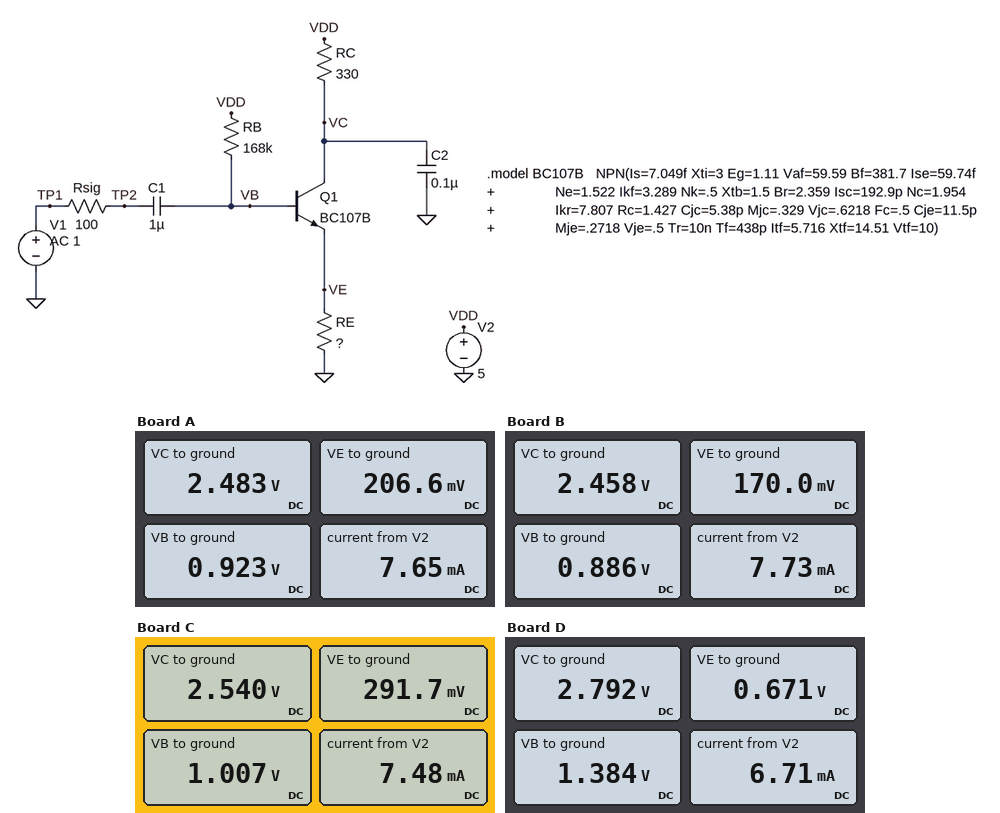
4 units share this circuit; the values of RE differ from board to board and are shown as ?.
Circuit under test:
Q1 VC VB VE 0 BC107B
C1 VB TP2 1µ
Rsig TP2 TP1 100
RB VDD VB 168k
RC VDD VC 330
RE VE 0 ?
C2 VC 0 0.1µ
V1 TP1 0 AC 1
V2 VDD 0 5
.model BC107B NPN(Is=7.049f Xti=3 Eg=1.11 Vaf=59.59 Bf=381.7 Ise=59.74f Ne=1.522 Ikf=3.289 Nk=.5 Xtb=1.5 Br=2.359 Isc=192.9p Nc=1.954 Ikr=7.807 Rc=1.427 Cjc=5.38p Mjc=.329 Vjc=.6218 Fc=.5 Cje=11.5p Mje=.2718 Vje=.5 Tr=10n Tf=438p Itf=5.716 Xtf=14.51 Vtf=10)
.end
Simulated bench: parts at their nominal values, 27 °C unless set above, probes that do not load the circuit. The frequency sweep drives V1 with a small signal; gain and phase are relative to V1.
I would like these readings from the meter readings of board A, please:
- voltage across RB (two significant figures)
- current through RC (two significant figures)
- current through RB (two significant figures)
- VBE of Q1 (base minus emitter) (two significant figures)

4.1 V
7.6 mA
24 µA
720 mV
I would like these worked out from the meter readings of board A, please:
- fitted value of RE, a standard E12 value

27 Ω
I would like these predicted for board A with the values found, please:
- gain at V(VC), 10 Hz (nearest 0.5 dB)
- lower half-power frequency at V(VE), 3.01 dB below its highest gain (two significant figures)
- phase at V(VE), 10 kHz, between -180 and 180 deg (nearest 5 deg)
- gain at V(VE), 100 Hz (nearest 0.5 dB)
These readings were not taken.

14.5 dB
17 Hz
0 deg
-1.5 dB
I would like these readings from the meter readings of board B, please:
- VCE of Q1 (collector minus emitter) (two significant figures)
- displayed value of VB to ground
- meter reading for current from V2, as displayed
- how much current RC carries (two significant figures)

2.3 V
0.886 V
7.73 mA
7.7 mA
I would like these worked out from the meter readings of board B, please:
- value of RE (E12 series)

22 Ω
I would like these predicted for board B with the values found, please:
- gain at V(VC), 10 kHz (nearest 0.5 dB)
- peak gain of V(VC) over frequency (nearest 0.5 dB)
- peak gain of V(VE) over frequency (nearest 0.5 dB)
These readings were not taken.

15.0 dB
22.0 dB
-1.5 dB
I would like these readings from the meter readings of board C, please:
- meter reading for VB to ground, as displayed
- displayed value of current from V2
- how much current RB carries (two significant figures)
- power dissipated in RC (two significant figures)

1.007 V
7.48 mA
24 µA
18 mW
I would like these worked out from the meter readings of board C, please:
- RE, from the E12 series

39 Ω
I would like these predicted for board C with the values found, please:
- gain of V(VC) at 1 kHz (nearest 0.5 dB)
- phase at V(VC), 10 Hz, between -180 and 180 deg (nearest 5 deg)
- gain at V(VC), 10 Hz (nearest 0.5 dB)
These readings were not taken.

17.5 dB
-130 deg
13.5 dB
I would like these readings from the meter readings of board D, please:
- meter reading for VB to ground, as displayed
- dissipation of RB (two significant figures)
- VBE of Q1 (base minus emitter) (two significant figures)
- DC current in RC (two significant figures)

1.384 V
78 µW
710 mV
6.7 mA
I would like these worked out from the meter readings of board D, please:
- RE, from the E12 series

100 Ω
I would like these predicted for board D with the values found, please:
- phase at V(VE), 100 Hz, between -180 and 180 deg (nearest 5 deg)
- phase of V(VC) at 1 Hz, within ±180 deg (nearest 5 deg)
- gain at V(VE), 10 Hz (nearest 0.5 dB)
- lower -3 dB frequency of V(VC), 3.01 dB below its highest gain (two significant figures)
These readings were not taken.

5 deg
-100 deg
-1.5 dB
5.7 Hz
